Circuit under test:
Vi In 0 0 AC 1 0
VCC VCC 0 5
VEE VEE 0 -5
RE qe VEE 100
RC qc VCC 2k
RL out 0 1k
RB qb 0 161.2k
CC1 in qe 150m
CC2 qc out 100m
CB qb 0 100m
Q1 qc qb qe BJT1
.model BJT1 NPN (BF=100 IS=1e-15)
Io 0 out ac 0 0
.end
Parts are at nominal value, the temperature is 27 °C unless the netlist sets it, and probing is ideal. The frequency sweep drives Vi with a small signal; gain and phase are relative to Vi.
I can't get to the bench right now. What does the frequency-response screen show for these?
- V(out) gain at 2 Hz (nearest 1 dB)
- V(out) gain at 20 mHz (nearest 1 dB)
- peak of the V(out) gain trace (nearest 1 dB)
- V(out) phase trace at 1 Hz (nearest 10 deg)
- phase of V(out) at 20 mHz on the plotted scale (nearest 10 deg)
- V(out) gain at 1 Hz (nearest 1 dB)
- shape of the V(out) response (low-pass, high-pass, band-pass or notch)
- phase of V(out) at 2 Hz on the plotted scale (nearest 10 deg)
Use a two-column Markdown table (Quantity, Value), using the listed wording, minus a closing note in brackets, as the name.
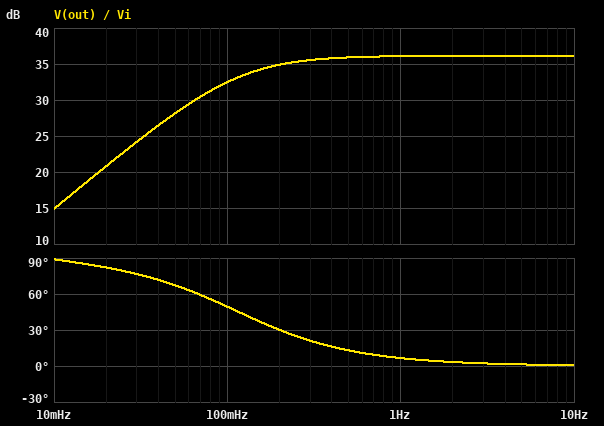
| Quantity | Value |
|---|---|
| V(out) gain at 2 Hz | 36 dB |
| V(out) gain at 20 mHz | 21 dB |
| peak of the V(out) gain trace | 36 dB |
| V(out) phase trace at 1 Hz | 10 deg |
| phase of V(out) at 20 mHz on the plotted scale | 80 deg |
| V(out) gain at 1 Hz | 36 dB |
| shape of the V(out) response | high-pass |
| phase of V(out) at 2 Hz on the plotted scale | 0 deg |
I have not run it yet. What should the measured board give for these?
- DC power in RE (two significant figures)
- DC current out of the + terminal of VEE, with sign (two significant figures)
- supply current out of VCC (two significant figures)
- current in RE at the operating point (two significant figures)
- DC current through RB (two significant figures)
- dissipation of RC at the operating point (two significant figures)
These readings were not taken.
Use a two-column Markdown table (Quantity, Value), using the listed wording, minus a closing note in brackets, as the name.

| Quantity | Value |
|---|---|
| DC power in RE | 630 µW |
| DC current out of the + terminal of VEE, with sign | -2.5 mA |
| supply current out of VCC | 2.5 mA |
| current in RE at the operating point | 2.5 mA |
| DC current through RB | 25 µA |
| dissipation of RC at the operating point | 12 mW |
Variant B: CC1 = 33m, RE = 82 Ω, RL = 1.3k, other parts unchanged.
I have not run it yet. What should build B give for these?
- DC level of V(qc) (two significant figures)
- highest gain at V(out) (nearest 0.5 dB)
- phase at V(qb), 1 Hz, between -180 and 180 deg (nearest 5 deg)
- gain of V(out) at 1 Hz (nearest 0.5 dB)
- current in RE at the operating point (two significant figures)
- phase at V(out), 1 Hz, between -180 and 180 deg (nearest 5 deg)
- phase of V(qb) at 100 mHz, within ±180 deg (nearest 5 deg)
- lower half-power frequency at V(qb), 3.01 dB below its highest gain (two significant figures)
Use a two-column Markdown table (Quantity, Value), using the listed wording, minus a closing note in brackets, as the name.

| Quantity | Value |
|---|---|
| DC level of V(qc) | -29 mV |
| highest gain at V(out) | 37.5 dB |
| phase at V(qb), 1 Hz, between -180 and 180 deg | -60 deg |
| gain of V(out) at 1 Hz | 36.5 dB |
| current in RE at the operating point | 2.5 mA |
| phase at V(out), 1 Hz, between -180 and 180 deg | 30 deg |
| phase of V(qb) at 100 mHz, within ±180 deg | -10 deg |
| lower half-power frequency at V(qb), 3.01 dB below its highest gain | 180 µHz |
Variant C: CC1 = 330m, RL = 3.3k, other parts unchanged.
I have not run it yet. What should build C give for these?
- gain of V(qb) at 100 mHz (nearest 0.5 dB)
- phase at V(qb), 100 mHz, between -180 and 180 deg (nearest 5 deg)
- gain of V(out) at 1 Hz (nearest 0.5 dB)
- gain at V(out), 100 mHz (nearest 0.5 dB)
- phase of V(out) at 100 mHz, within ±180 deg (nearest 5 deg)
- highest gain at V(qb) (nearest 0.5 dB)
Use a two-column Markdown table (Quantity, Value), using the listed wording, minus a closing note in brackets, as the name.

| Quantity | Value |
|---|---|
| gain of V(qb) at 100 mHz | -37.5 dB |
| phase at V(qb), 100 mHz, between -180 and 180 deg | -60 deg |
| gain of V(out) at 1 Hz | 41.5 dB |
| gain at V(out), 100 mHz | 40.5 dB |
| phase of V(out) at 100 mHz, within ±180 deg | 30 deg |
| highest gain at V(qb) | -31.0 dB |
